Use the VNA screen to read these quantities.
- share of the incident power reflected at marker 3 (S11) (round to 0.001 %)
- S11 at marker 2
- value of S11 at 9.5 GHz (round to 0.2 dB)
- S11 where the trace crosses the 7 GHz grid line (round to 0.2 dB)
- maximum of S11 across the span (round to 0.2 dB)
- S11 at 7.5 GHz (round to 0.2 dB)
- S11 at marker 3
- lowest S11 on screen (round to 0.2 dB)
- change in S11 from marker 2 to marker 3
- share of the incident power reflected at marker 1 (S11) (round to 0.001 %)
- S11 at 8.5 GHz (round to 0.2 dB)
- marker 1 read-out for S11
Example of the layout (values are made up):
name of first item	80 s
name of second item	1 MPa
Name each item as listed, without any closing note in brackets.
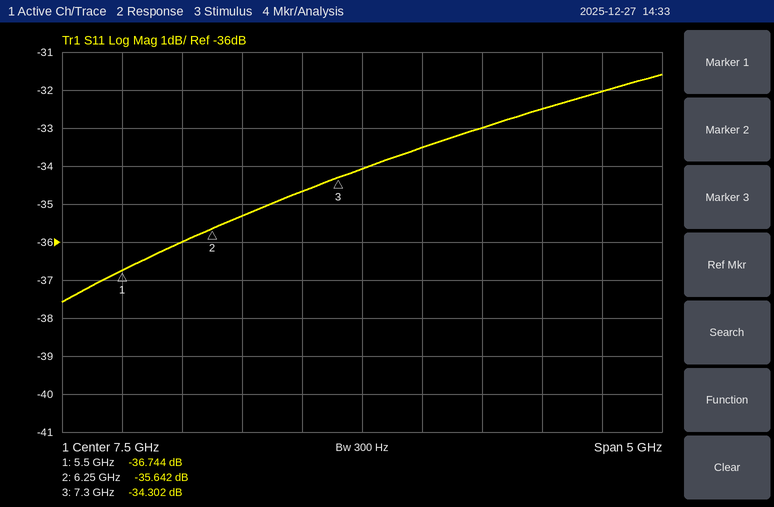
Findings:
share of the incident power reflected at marker 3 (S11)	0.037 %
S11 at marker 2	-35.642 dB
value of S11 at 9.5 GHz	-32.0 dB
S11 where the trace crosses the 7 GHz grid line	-34.6 dB
maximum of S11 across the span	-31.6 dB
S11 at 7.5 GHz	-34.0 dB
S11 at marker 3	-34.302 dB
lowest S11 on screen	-37.6 dB
change in S11 from marker 2 to marker 3	1.340 dB
share of the incident power reflected at marker 1 (S11)	0.021 %
S11 at 8.5 GHz	-33.0 dB
marker 1 read-out for S11	-36.744 dB
